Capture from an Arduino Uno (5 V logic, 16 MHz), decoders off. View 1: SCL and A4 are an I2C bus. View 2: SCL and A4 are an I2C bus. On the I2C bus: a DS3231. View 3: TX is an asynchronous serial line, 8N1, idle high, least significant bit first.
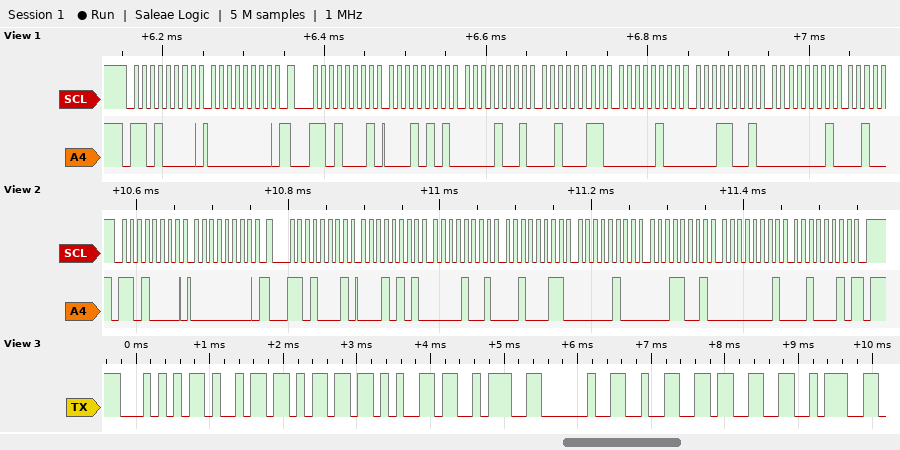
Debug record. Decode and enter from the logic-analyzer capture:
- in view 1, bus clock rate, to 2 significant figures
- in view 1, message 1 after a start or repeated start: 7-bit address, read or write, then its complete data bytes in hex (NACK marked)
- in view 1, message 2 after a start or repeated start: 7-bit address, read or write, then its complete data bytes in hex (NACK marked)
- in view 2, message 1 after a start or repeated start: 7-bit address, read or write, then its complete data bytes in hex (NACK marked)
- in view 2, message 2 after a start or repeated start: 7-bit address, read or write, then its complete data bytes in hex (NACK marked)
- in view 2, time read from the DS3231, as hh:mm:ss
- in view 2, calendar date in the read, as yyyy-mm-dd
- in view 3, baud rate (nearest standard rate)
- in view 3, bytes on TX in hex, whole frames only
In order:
100 kHz
0x68 write: 00
0x68 read: 15 09 23 04 19 01
0x68 write: 00
0x68 read: 15 09 23 04 19 01 22 NACK
23:09:15
2022-01-19
9600 baud
0x54 0x69 0x6D 0x65 0x3A 0x20 0x32 0x33 0x3A
